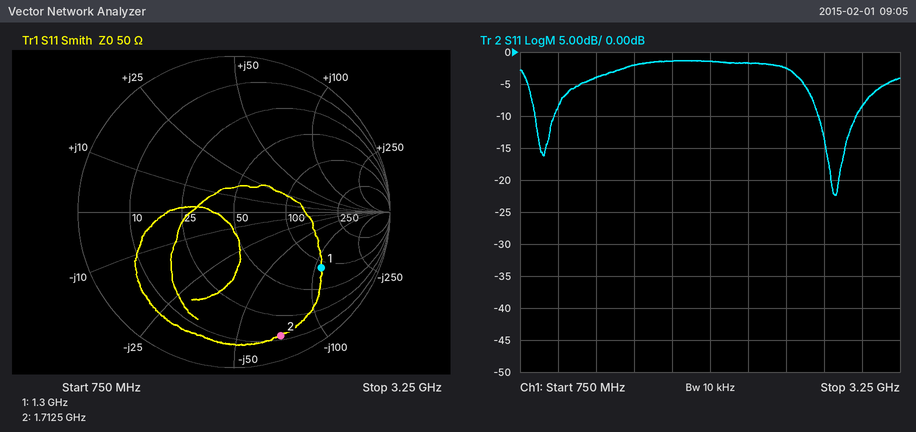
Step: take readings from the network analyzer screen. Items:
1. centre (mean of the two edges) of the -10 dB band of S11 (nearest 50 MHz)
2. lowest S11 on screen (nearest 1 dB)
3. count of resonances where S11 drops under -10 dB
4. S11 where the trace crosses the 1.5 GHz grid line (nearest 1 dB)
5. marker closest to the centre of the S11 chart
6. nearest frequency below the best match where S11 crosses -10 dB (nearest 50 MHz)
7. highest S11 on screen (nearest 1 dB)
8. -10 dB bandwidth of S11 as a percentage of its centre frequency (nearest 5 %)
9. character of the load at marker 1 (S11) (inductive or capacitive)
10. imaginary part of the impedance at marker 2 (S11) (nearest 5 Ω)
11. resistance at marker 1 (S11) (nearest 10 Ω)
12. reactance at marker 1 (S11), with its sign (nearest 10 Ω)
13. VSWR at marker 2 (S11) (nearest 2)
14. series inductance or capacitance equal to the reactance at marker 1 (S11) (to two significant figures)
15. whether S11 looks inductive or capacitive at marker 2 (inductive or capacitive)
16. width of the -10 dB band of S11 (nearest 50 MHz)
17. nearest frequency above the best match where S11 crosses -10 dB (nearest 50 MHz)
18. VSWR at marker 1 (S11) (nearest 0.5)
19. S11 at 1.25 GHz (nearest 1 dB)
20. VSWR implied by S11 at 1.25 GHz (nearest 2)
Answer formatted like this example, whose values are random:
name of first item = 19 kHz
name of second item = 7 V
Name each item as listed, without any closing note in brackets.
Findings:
centre (mean of the two edges) of the -10 dB band of S11 = 2.85 GHz
lowest S11 on screen = -22 dB
count of resonances where S11 drops under -10 dB = 2
S11 where the trace crosses the 1.5 GHz grid line = -2 dB
marker closest to the centre of the S11 chart = marker 1
nearest frequency below the best match where S11 crosses -10 dB = 2.70 GHz
highest S11 on screen = -1 dB
-10 dB bandwidth of S11 as a percentage of its centre frequency = 10 %
character of the load at marker 1 (S11) = capacitive
imaginary part of the impedance at marker 2 (S11) = -70 Ω
resistance at marker 1 (S11) = 90 Ω
reactance at marker 1 (S11), with its sign = -110 Ω
VSWR at marker 2 (S11) = 12
series inductance or capacitance equal to the reactance at marker 1 (S11) = 1.1 pF
whether S11 looks inductive or capacitive at marker 2 = capacitive
width of the -10 dB band of S11 = 250 MHz
nearest frequency above the best match where S11 crosses -10 dB = 2.95 GHz
VSWR at marker 1 (S11) = 5.0
S11 at 1.25 GHz = -4 dB
VSWR implied by S11 at 1.25 GHz = 4
